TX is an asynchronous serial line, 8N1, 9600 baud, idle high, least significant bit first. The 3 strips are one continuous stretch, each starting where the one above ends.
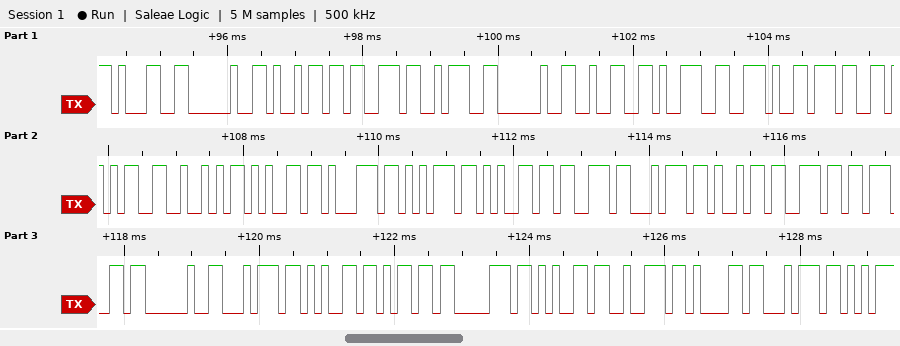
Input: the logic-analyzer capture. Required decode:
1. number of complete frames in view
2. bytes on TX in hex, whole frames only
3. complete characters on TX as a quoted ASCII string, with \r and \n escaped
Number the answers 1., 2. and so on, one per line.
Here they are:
1. 30
2. 31 20 69 73 3A 20 32 39 2E 37 35 52 65 71 75 65 73 74 69 6E 67 20 74 65 6D 70 65 72 61 74
3. "1 is: 29.75Requesting temperat"
